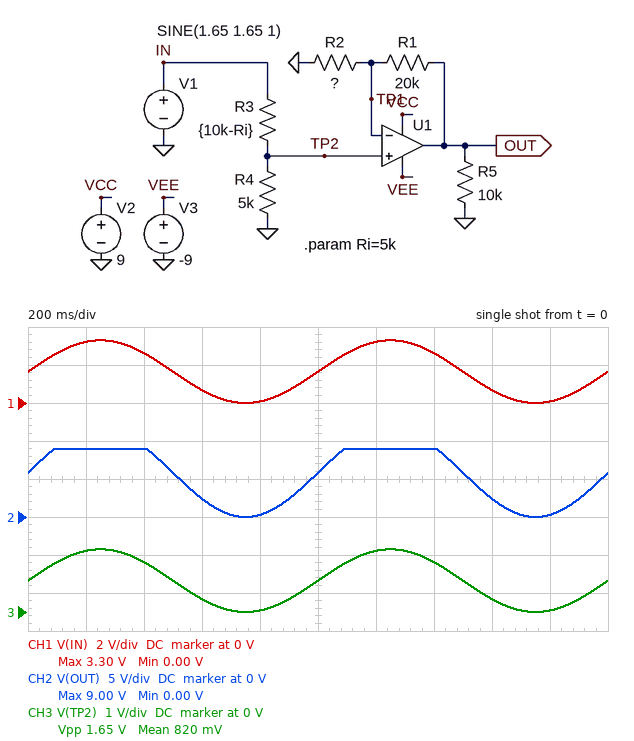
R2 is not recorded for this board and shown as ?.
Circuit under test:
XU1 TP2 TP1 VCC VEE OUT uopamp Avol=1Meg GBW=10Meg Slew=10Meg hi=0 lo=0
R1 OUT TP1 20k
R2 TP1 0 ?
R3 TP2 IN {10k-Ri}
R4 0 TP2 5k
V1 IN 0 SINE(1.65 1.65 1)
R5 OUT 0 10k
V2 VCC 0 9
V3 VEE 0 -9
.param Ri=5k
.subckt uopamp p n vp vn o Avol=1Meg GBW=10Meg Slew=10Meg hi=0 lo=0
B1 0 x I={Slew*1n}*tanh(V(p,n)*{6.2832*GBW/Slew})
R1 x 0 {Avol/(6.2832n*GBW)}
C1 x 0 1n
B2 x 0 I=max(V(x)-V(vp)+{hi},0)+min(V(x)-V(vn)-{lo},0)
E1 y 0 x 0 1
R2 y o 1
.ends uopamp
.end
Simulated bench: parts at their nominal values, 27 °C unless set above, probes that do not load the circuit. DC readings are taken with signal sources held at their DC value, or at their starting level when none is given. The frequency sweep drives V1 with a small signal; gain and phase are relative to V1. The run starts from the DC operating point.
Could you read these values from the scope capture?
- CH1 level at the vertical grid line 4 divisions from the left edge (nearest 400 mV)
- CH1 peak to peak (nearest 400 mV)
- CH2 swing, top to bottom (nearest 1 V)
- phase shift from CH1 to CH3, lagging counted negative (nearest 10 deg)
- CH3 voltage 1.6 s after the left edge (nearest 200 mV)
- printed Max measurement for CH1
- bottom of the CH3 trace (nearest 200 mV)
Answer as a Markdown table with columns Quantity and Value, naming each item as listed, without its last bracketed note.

| Quantity | Value |
|---|---|
| CH1 level at the vertical grid line 4 divisions from the left edge | 0 V |
| CH1 peak to peak | 3.2 V |
| CH2 swing, top to bottom | 9 V |
| phase shift from CH1 to CH3, lagging counted negative | 0 deg |
| CH3 voltage 1.6 s after the left edge | 400 mV |
| printed Max measurement for CH1 | 3.30 V |
| bottom of the CH3 trace | 0 V |
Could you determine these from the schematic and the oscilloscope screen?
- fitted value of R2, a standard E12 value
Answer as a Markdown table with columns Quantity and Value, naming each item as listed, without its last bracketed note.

| Quantity | Value |
|---|---|
| fitted value of R2, a standard E12 value | 3.3 kΩ |
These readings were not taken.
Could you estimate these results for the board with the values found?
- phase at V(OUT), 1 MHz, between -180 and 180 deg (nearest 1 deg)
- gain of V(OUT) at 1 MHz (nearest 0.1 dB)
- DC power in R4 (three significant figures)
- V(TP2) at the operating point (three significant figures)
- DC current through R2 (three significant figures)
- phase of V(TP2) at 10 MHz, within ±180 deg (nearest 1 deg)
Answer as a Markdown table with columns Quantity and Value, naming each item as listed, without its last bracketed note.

| Quantity | Value |
|---|---|
| phase at V(OUT), 1 MHz, between -180 and 180 deg | -35 deg |
| gain of V(OUT) at 1 MHz | 9.2 dB |
| DC power in R4 | 136 µW |
| V(TP2) at the operating point | 825 mV |
| DC current through R2 | 250 µA |
| phase of V(TP2) at 10 MHz, within ±180 deg | 0 deg |
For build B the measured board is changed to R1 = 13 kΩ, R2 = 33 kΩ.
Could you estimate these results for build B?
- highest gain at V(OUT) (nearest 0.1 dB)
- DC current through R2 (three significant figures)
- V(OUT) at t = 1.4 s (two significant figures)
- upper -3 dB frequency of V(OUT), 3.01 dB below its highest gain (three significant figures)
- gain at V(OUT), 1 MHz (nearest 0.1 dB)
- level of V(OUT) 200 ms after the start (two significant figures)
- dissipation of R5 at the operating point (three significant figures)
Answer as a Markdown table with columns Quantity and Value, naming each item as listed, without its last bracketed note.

| Quantity | Value |
|---|---|
| highest gain at V(OUT) | -3.1 dB |
| DC current through R2 | 25.0 µA |
| V(OUT) at t = 1.4 s | 1.8 V |
| upper -3 dB frequency of V(OUT), 3.01 dB below its highest gain | 7.17 MHz |
| gain at V(OUT), 1 MHz | -3.2 dB |
| level of V(OUT) 200 ms after the start | 2.2 V |
| dissipation of R5 at the operating point | 132 µW |
